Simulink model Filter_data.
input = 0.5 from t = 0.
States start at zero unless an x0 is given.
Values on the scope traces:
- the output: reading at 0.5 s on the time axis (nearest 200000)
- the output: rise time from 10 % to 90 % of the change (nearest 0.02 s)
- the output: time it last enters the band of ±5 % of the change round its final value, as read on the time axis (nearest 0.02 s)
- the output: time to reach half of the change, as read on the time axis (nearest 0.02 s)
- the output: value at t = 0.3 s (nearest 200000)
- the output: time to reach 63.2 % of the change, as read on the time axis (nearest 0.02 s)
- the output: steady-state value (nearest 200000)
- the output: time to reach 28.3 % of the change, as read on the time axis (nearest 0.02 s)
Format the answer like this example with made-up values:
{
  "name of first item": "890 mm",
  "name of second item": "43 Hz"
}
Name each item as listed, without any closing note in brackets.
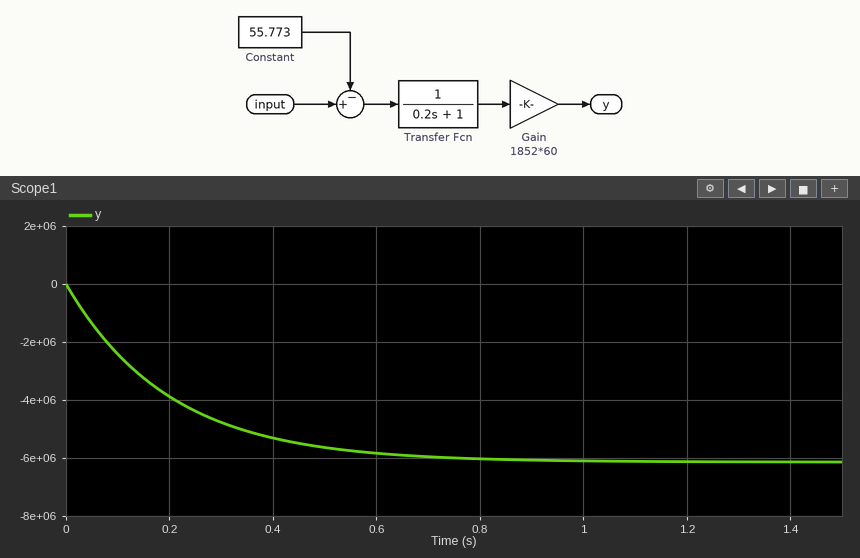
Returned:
{
  "the output: reading at 0.5 s on the time axis": "-5600000",
  "the output: rise time from 10 % to 90 % of the change": "0.44 s",
  "the output: time it last enters the band of ±5 % of the change round its final value, as read on the time axis": "0.60 s",
  "the output: time to reach half of the change, as read on the time axis": "0.14 s",
  "the output: value at t = 0.3 s": "-4800000",
  "the output: time to reach 63.2 % of the change, as read on the time axis": "0.20 s",
  "the output: steady-state value": "-6200000",
  "the output: time to reach 28.3 % of the change, as read on the time axis": "0.06 s"
}
